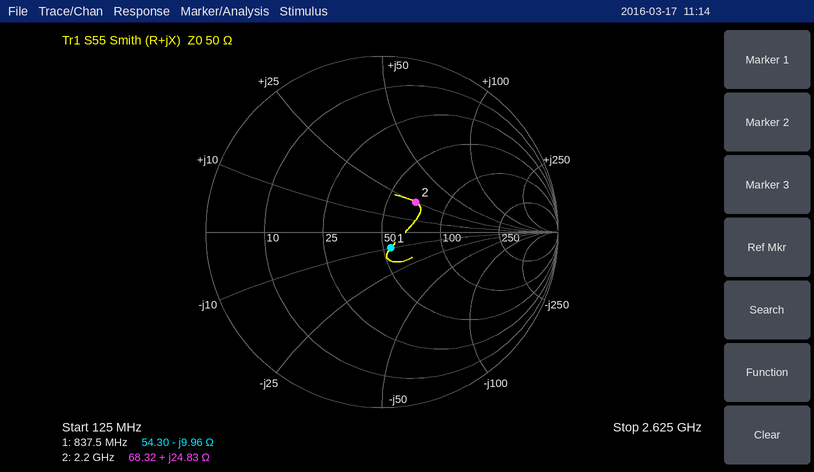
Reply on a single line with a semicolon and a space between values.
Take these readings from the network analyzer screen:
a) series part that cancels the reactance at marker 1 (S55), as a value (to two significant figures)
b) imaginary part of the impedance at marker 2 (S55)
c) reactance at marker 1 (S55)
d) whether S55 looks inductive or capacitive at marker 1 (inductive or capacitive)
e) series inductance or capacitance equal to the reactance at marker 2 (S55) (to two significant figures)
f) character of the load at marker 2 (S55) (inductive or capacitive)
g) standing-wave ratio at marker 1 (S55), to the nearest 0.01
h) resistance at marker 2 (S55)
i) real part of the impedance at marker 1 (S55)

1.9 nH; +24.83 Ω; -9.96 Ω; capacitive; 1.8 nH; inductive; 1.23; 68.32 Ω; 54.30 Ω
